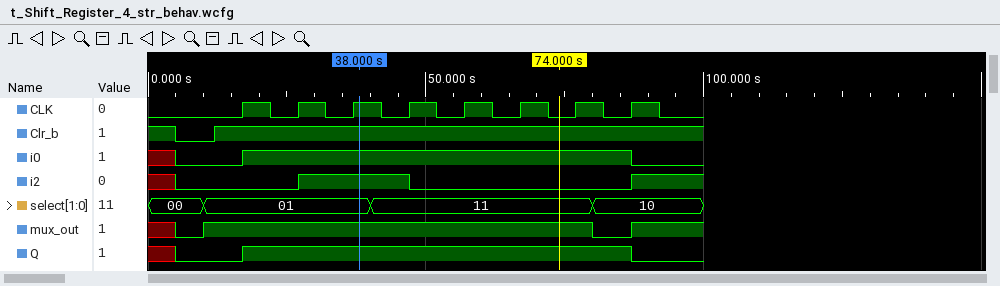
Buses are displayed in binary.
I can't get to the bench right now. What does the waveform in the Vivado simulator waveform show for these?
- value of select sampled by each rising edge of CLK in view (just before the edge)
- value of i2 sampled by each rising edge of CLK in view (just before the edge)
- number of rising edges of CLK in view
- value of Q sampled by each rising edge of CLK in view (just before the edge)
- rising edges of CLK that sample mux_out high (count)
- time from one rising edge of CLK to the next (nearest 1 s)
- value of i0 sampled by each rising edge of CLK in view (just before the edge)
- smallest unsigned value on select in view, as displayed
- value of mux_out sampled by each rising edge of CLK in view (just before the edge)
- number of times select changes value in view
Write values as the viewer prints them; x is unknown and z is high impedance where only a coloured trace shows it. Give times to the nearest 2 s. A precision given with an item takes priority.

01, 01, 01, 11, 11, 11, 11, 10
0 0 1 1 0 0 0 0
8
0 1 1 1 1 1 1 1
7
10 s
0 1 1 1 1 1 1 1
00
1 1 1 1 1 1 1 0
3
